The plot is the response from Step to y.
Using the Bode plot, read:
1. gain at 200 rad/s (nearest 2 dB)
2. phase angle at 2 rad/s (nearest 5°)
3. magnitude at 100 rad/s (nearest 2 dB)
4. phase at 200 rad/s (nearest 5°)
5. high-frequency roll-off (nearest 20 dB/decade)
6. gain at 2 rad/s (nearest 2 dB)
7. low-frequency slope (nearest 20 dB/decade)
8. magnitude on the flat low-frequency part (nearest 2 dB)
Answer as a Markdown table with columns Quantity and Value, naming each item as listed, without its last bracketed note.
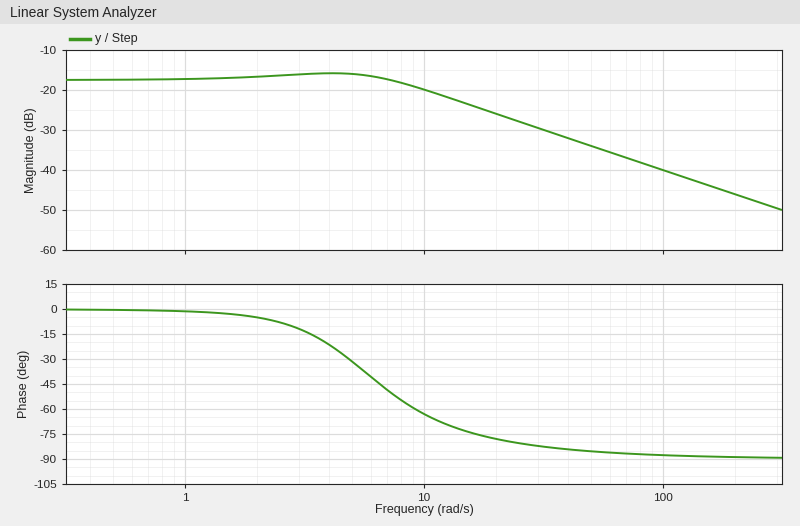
| Quantity | Value |
|---|---|
| gain at 200 rad/s | -46 dB |
| phase angle at 2 rad/s | -5° |
| magnitude at 100 rad/s | -40 dB |
| phase at 200 rad/s | -90° |
| high-frequency roll-off | -20 dB/decade |
| gain at 2 rad/s | -16 dB |
| low-frequency slope | 0 dB/decade |
| magnitude on the flat low-frequency part | -18 dB |
